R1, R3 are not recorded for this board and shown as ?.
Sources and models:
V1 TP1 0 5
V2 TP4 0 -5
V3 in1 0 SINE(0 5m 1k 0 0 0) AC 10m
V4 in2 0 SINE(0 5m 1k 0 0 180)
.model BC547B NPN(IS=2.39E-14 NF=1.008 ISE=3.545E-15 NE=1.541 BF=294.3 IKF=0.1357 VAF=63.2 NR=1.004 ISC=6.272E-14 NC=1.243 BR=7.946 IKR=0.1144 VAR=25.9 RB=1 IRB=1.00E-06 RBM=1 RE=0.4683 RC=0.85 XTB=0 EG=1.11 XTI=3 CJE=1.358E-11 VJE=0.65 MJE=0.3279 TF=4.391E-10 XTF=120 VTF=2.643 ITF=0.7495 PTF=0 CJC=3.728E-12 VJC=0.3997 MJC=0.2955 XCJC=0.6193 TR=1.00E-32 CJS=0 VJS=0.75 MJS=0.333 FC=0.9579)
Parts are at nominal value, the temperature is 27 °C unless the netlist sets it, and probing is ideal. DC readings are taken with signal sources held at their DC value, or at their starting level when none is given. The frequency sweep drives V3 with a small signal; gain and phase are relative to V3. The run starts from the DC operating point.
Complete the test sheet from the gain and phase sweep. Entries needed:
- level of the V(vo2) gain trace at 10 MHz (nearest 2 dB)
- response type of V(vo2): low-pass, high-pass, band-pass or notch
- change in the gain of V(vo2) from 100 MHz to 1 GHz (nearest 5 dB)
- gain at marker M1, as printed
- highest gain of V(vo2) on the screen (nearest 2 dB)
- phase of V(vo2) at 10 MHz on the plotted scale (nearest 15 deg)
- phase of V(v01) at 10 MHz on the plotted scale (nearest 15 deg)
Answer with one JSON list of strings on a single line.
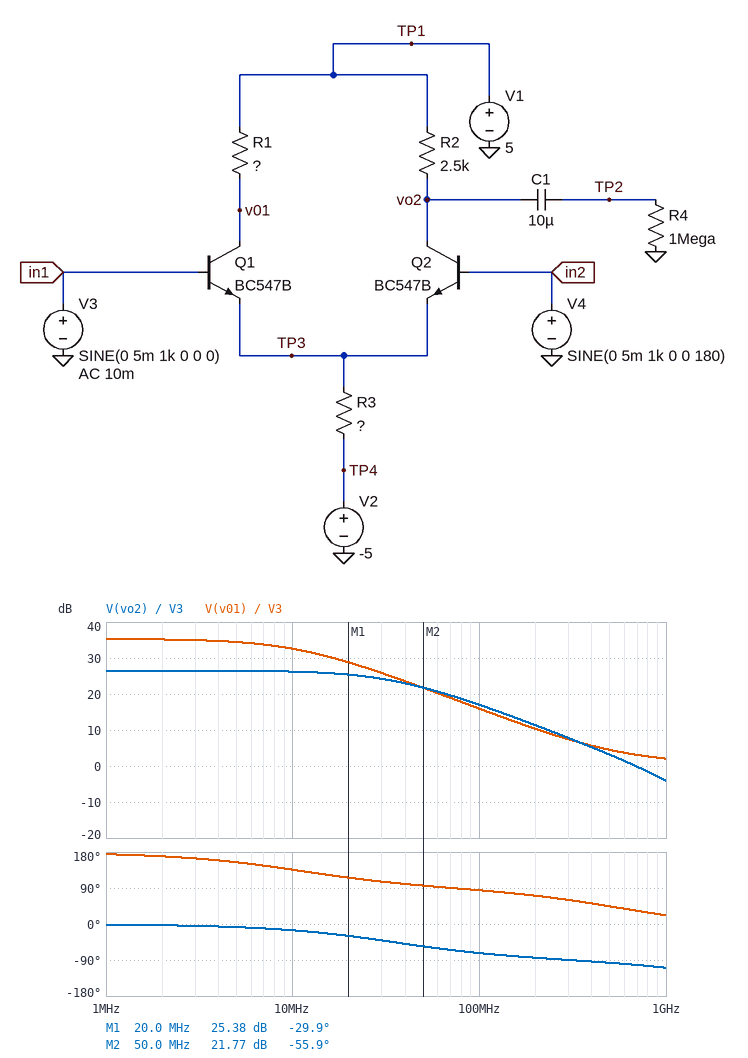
["26 dB", "low-pass", "-20 dB", "25.38 dB", "26 dB", "-15 deg", "135 deg"]
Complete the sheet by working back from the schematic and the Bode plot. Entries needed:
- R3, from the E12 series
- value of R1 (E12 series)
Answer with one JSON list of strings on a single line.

["4.7 kΩ", "6.8 kΩ"]
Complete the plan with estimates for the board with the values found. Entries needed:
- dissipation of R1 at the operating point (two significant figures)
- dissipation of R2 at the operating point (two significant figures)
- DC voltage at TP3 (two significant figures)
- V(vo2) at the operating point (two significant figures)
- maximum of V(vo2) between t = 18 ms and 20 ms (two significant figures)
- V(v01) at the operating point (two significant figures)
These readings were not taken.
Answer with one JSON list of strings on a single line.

["1.4 mW", "560 µW", "-620 mV", "3.8 V", "4.0 V", "1.9 V"]
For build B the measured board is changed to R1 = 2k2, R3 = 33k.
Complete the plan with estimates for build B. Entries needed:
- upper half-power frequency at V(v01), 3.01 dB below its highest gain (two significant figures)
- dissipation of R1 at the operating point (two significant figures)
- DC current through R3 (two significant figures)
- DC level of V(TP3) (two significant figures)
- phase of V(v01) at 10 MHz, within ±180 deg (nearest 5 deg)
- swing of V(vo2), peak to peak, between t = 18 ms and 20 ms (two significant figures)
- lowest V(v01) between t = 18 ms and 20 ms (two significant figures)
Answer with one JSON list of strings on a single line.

["48 MHz", "9.9 µW", "130 µA", "-570 mV", "160 deg", "63 mV", "4.8 V"]
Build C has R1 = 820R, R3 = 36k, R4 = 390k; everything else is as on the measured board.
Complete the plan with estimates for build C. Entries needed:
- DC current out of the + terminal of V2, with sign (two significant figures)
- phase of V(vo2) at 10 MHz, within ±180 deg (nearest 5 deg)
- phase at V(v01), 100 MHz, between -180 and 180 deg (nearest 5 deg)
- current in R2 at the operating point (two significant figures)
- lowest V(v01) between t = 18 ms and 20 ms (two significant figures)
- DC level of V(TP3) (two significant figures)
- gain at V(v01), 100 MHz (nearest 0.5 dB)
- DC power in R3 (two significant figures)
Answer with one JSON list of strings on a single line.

["-120 µA", "-15 deg", "95 deg", "61 µA", "4.9 V", "-560 mV", "0 dB", "550 µW"]
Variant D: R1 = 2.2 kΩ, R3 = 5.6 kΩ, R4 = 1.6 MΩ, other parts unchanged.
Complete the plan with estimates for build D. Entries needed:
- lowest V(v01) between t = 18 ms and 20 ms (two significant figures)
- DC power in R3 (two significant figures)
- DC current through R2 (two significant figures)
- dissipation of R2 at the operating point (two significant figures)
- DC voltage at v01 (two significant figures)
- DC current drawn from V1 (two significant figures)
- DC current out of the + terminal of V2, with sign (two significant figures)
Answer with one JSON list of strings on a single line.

["4.0 V", "3.4 mW", "390 µA", "380 µW", "4.1 V", "780 µA", "-780 µA"]
